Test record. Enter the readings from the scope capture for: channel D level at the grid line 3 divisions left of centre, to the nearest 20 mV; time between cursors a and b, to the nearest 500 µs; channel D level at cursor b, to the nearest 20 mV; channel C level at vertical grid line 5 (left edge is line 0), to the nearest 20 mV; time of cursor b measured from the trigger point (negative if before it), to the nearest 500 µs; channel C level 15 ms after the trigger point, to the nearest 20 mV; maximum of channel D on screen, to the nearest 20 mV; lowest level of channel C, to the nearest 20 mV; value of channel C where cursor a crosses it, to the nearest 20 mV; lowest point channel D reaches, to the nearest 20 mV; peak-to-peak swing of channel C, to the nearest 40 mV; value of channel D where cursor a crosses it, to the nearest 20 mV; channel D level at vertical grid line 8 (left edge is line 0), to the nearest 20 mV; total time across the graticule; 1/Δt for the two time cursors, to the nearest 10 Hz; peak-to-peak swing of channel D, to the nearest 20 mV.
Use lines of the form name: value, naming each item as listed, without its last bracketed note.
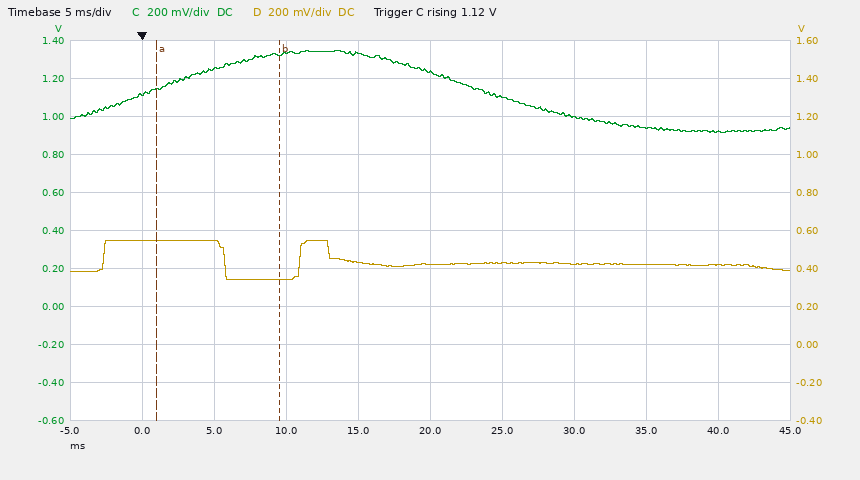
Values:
channel D level at the grid line 3 divisions left of centre, to the nearest 20 mV: 540 mV
time between cursors a and b, to the nearest 500 µs: 8.5 ms
channel D level at cursor b, to the nearest 20 mV: 340 mV
channel C level at vertical grid line 5 (left edge is line 0), to the nearest 20 mV: 1.24 V
time of cursor b measured from the trigger point (negative if before it), to the nearest 500 µs: +9.5 ms
channel C level 15 ms after the trigger point, to the nearest 20 mV: 1.34 V
maximum of channel D on screen, to the nearest 20 mV: 540 mV
lowest level of channel C, to the nearest 20 mV: 920 mV
value of channel C where cursor a crosses it, to the nearest 20 mV: 1.14 V
lowest point channel D reaches, to the nearest 20 mV: 340 mV
peak-to-peak swing of channel C, to the nearest 40 mV: 440 mV
value of channel D where cursor a crosses it, to the nearest 20 mV: 540 mV
channel D level at vertical grid line 8 (left edge is line 0), to the nearest 20 mV: 420 mV
total time across the graticule: 50 ms
1/Δt for the two time cursors, to the nearest 10 Hz: 120 Hz
peak-to-peak swing of channel D, to the nearest 20 mV: 200 mV
